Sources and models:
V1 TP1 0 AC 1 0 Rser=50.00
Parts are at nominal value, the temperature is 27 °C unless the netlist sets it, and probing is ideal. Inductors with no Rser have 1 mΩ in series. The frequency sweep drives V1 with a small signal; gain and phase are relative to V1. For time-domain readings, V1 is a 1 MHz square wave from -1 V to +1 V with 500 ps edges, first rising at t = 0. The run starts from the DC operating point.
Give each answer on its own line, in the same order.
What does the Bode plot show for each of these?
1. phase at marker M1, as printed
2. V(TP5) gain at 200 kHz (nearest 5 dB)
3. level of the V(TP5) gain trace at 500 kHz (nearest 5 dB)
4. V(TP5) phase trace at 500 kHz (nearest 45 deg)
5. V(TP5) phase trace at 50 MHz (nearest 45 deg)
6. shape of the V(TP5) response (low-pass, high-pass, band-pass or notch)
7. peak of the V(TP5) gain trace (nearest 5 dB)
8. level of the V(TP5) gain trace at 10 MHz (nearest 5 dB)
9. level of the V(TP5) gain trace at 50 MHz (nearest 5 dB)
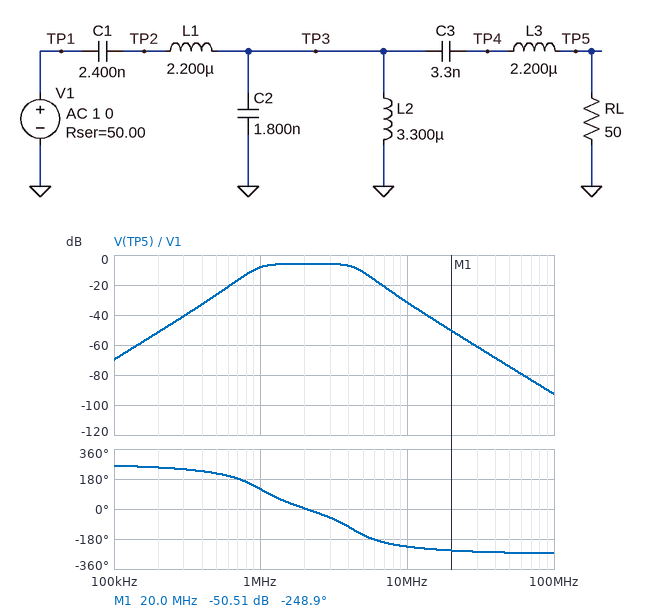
-248.9 deg
-50 dB
-25 dB
225 deg
-270 deg
band-pass
-5 dB
-30 dB
-75 dB
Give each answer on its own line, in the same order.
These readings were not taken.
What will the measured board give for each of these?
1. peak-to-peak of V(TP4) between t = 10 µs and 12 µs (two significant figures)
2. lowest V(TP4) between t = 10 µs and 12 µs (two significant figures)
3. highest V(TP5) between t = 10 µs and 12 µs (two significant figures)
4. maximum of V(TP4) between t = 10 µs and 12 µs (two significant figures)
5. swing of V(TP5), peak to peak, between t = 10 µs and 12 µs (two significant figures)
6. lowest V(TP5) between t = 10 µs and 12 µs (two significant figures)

1.3 V
-630 mV
550 mV
630 mV
1.1 V
-550 mV
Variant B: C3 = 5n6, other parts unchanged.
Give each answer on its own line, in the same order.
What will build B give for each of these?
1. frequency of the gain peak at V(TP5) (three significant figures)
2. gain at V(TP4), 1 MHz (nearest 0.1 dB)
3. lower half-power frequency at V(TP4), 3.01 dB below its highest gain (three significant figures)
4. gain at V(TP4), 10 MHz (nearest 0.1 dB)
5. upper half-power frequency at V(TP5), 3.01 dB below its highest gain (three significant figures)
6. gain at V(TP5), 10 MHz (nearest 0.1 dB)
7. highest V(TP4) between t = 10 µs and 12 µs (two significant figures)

2.67 MHz
-8.2 dB
1.21 MHz
-22.4 dB
4.46 MHz
-31.8 dB
660 mV
